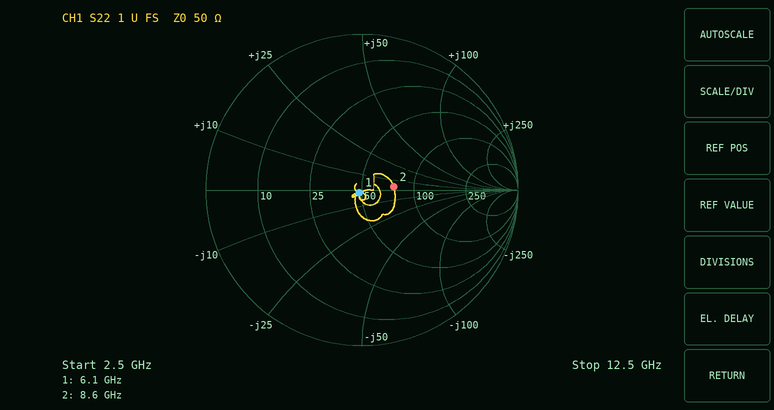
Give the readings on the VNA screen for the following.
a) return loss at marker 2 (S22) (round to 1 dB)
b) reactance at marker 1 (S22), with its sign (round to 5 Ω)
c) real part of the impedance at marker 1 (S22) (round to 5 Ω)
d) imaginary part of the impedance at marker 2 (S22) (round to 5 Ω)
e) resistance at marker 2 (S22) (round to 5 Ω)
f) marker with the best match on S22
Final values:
14 dB
0 Ω
50 Ω
+5 Ω
75 Ω
marker 1
